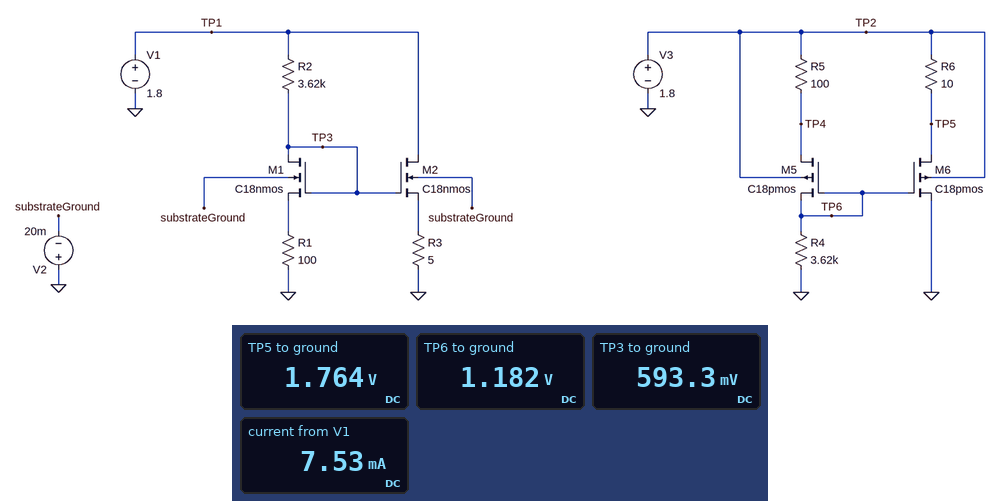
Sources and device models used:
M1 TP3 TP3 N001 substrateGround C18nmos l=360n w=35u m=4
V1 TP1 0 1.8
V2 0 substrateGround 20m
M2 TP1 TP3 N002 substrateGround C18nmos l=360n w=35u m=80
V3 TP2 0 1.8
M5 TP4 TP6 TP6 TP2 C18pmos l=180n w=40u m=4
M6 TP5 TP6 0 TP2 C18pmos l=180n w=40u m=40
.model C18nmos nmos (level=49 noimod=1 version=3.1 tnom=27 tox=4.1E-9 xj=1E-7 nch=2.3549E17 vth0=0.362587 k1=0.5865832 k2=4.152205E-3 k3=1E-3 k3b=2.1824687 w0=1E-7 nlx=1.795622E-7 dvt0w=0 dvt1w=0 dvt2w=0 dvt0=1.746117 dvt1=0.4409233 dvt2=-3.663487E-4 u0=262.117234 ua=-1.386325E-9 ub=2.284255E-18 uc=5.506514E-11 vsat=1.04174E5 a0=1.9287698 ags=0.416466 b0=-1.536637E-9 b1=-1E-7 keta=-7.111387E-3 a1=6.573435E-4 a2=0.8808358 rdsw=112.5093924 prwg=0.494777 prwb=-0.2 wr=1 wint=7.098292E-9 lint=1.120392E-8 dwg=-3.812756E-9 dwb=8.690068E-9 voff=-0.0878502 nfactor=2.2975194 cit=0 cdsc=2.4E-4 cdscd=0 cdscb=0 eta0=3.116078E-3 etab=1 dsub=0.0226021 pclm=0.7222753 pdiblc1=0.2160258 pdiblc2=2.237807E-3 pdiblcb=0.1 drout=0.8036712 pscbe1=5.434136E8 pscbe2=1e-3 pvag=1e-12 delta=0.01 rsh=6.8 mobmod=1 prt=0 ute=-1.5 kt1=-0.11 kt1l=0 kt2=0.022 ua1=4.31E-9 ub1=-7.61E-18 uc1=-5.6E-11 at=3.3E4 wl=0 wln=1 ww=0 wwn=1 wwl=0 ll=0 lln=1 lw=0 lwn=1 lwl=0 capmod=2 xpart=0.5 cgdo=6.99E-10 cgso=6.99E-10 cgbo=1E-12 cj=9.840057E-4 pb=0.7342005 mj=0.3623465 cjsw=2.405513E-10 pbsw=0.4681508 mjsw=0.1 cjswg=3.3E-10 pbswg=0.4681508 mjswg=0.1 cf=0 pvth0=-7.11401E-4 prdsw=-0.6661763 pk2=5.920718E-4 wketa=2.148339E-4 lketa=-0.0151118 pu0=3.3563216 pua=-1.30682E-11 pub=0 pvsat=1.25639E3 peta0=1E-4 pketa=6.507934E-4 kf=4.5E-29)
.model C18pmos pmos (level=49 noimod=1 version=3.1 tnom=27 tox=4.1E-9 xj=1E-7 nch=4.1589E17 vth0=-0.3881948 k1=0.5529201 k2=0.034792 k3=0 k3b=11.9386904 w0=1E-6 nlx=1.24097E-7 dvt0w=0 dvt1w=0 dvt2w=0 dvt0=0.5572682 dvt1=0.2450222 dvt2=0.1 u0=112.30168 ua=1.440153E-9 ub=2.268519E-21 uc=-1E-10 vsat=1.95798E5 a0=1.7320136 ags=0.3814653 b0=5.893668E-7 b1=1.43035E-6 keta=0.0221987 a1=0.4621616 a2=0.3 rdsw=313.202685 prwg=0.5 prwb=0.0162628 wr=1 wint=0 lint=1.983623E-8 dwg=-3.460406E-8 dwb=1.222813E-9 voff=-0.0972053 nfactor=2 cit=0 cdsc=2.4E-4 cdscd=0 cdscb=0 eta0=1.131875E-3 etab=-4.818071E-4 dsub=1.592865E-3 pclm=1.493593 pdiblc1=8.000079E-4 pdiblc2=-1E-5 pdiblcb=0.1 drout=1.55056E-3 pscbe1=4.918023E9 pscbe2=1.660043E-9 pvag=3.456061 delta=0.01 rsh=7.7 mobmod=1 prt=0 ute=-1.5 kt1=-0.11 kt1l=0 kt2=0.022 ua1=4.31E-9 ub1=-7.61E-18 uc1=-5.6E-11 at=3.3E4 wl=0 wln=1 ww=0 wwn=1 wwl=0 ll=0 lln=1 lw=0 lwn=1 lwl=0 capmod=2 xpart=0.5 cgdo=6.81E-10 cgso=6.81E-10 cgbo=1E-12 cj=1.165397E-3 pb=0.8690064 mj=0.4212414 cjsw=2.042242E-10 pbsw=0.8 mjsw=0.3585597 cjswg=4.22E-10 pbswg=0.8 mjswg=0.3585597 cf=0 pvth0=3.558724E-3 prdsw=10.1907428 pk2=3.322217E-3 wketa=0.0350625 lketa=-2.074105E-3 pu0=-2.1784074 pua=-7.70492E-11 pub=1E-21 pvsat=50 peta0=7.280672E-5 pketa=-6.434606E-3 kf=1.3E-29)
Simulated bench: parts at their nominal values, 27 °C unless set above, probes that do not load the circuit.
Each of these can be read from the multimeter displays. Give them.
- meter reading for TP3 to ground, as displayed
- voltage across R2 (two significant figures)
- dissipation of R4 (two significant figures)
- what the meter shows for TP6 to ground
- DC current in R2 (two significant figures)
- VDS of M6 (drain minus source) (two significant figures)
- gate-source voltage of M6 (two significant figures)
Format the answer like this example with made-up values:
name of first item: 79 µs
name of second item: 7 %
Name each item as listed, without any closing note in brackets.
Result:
meter reading for TP3 to ground, as displayed: 593.3 mV
voltage across R2: 1.2 V
dissipation of R4: 390 µW
what the meter shows for TP6 to ground: 1.182 V
DC current in R2: 330 µA
VDS of M6 (drain minus source): 1.8 V
gate-source voltage of M6: 1.2 V
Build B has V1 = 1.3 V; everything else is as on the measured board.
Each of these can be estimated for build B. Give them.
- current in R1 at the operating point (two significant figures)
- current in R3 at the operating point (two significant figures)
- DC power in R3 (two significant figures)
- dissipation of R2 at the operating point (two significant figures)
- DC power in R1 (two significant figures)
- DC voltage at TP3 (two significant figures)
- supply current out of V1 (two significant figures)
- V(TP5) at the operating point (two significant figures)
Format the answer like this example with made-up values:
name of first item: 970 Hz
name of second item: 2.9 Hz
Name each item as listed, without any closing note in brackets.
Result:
current in R1 at the operating point: 210 µA
current in R3 at the operating point: 4.3 mA
DC power in R3: 92 µW
dissipation of R2 at the operating point: 150 µW
DC power in R1: 4.3 µW
DC voltage at TP3: 550 mV
supply current out of V1: 4.5 mA
V(TP5) at the operating point: 1.8 V
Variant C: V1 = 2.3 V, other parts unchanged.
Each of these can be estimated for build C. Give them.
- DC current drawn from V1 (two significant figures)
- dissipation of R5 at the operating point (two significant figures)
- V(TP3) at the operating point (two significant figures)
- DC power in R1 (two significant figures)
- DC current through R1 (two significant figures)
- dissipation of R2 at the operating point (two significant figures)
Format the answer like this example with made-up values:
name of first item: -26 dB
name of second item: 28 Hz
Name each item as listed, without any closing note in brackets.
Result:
DC current drawn from V1: 13 mA
dissipation of R5 at the operating point: 11 µW
V(TP3) at the operating point: 630 mV
DC power in R1: 21 µW
DC current through R1: 460 µA
dissipation of R2 at the operating point: 770 µW
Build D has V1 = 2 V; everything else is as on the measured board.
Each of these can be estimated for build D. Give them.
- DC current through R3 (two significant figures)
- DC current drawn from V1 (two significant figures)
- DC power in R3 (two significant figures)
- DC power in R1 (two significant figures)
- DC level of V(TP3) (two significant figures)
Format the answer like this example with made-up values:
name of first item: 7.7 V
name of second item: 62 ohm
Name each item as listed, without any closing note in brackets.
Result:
DC current through R3: 8.9 mA
DC current drawn from V1: 9.3 mA
DC power in R3: 390 µW
DC power in R1: 15 µW
DC level of V(TP3): 610 mV
